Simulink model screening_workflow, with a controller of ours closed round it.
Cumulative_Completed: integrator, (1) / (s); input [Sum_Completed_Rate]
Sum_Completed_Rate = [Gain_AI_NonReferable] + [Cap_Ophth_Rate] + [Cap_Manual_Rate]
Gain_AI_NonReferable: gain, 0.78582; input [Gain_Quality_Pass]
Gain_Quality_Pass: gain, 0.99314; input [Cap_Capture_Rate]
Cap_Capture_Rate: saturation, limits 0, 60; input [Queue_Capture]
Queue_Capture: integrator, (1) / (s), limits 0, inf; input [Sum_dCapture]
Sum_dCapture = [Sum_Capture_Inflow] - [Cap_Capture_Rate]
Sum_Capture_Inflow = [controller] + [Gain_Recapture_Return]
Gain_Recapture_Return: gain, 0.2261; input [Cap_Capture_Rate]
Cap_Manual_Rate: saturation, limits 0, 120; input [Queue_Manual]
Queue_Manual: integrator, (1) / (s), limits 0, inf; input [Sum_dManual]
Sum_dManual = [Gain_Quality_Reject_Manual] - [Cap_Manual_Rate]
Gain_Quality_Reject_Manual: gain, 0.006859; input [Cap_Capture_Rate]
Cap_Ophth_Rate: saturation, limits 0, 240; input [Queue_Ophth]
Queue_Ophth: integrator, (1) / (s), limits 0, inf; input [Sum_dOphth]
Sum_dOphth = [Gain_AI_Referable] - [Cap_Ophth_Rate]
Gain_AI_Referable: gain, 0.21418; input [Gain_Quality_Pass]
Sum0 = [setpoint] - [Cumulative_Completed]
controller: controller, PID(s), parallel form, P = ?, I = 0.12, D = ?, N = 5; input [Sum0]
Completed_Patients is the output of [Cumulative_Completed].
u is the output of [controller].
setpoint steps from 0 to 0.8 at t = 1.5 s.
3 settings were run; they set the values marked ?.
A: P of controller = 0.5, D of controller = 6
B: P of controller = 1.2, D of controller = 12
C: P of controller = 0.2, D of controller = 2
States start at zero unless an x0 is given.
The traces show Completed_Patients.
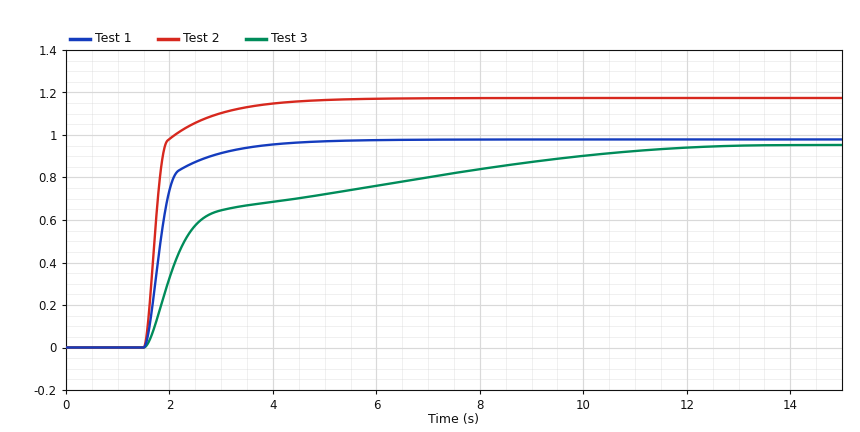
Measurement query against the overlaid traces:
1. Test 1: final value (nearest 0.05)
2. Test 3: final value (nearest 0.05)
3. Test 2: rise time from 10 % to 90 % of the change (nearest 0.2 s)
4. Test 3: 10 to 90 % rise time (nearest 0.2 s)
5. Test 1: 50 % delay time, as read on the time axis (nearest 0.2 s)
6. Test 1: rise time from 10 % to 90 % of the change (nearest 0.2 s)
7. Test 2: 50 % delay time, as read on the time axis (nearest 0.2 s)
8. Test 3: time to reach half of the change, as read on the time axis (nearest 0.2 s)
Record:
1.00
0.95
1.0 s
6.8 s
1.8 s
1.0 s
1.8 s
2.2 s
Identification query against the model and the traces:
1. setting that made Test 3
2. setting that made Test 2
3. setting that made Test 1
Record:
C
B
A
